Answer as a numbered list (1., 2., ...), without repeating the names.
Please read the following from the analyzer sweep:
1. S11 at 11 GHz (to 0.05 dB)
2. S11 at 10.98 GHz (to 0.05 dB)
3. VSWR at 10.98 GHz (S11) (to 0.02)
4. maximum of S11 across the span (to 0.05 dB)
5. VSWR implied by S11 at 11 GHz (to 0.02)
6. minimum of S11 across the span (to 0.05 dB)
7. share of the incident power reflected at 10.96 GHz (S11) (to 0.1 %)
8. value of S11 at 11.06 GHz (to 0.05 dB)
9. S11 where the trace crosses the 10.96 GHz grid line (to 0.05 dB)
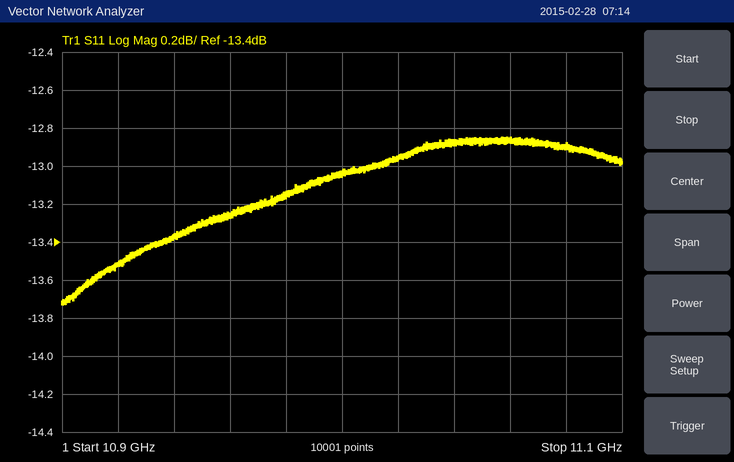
1. -13.05 dB
2. -13.15 dB
3. 1.56
4. -12.85 dB
5. 1.58
6. -13.75 dB
7. 4.7 %
8. -12.85 dB
9. -13.25 dB
